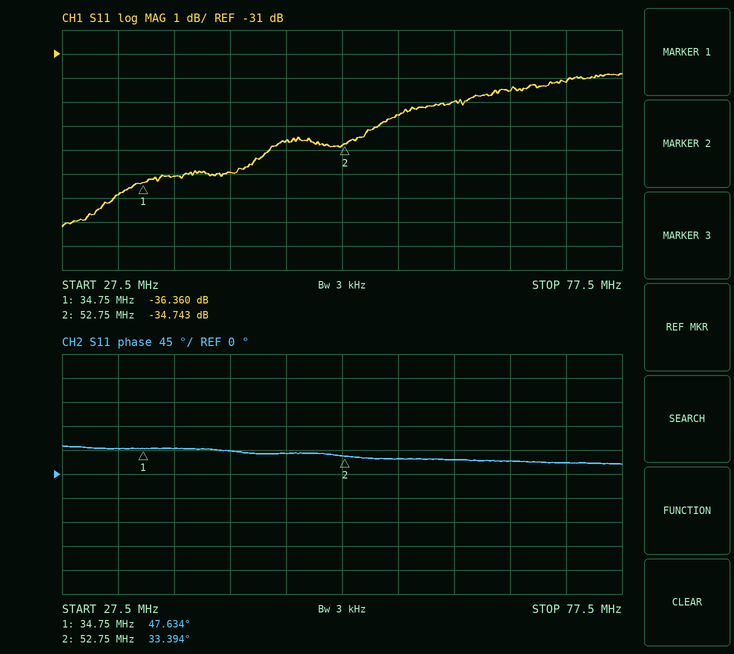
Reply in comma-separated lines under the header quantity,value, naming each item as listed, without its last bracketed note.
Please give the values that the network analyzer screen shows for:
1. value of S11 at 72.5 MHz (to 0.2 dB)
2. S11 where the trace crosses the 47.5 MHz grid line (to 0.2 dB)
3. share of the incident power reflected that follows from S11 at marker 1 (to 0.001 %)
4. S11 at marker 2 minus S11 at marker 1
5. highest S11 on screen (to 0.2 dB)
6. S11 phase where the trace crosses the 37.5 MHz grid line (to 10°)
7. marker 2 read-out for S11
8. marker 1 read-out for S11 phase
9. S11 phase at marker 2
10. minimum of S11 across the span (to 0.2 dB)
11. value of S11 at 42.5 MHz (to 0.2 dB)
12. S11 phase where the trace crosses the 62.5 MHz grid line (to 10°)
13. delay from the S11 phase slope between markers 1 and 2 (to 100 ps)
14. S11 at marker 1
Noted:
quantity,value
value of S11 at 72.5 MHz,-32.2 dB
S11 where the trace crosses the 47.5 MHz grid line,-34.6 dB
share of the incident power reflected that follows from S11 at marker 1,0.023 %
S11 at marker 2 minus S11 at marker 1,1.617 dB
highest S11 on screen,-31.8 dB
S11 phase where the trace crosses the 37.5 MHz grid line,50°
marker 2 read-out for S11,-34.743 dB
marker 1 read-out for S11 phase,47.634°
S11 phase at marker 2,33.394°
minimum of S11 across the span,-38.2 dB
value of S11 at 42.5 MHz,-36.0 dB
S11 phase where the trace crosses the 62.5 MHz grid line,30°
delay from the S11 phase slope between markers 1 and 2,2.2 ns
S11 at marker 1,-36.360 dB
